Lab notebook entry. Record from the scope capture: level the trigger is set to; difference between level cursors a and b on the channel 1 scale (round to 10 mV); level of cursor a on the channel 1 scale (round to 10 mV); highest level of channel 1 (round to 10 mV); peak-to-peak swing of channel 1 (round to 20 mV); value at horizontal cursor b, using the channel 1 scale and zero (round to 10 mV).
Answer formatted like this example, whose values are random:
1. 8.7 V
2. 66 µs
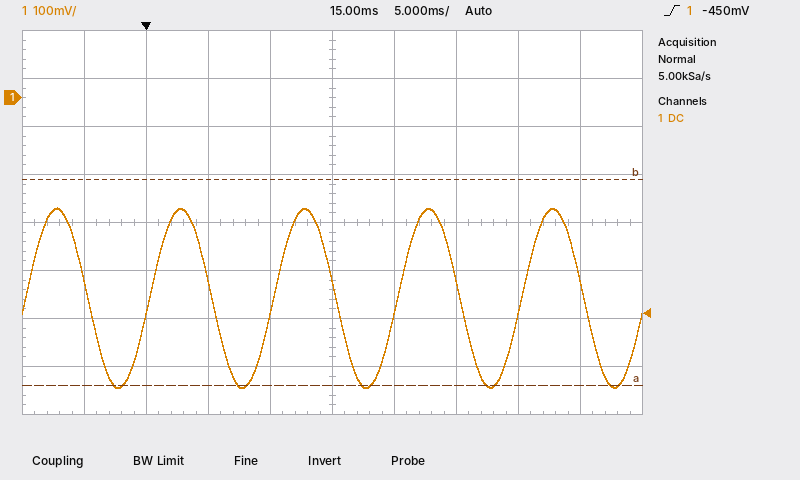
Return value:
1. -450 mV
2. 430 mV
3. -600 mV
4. -230 mV
5. 380 mV
6. -170 mV
